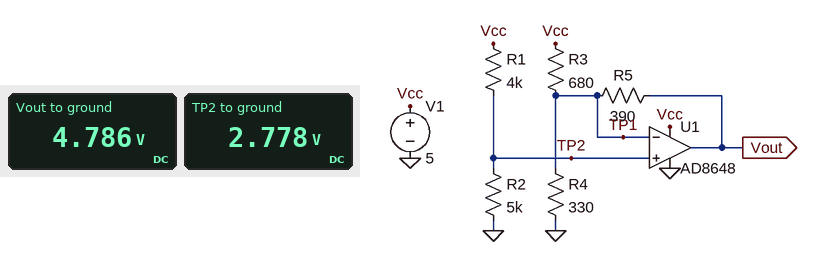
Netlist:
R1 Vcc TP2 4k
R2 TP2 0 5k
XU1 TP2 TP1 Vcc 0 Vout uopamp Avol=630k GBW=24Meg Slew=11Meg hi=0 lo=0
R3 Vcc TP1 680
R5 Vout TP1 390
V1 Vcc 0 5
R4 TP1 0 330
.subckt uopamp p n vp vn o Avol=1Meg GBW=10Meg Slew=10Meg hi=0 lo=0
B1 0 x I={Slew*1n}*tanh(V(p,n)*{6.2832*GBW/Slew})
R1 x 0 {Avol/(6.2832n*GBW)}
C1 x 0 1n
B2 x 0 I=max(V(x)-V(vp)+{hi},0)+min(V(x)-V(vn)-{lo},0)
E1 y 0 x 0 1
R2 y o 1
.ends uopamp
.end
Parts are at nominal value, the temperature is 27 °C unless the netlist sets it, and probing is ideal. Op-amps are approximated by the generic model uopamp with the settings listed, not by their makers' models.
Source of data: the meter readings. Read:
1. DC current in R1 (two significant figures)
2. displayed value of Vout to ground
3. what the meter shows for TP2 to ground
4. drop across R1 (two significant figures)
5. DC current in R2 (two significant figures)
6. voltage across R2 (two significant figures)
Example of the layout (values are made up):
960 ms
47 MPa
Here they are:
560 µA
4.786 V
2.778 V
2.2 V
560 µA
2.8 V
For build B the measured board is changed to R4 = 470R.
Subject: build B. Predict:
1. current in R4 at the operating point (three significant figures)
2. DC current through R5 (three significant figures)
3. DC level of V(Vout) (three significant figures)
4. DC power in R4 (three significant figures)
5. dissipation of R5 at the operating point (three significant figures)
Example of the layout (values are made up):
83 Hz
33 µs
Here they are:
5.91 mA
2.64 mA
3.81 V
16.4 mW
2.72 mW
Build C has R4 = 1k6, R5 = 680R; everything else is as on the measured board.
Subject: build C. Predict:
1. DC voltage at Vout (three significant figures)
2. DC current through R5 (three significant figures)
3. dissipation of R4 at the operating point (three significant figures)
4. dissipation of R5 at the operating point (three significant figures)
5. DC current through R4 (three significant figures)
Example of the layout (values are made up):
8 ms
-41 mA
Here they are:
1.74 V
1.53 mA
4.82 mW
1.60 mW
1.74 mA
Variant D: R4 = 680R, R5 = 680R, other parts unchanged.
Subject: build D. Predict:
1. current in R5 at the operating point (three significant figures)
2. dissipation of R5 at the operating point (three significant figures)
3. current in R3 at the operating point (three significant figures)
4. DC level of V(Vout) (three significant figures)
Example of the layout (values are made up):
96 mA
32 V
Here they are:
817 µA
454 µW
3.27 mA
3.33 V
